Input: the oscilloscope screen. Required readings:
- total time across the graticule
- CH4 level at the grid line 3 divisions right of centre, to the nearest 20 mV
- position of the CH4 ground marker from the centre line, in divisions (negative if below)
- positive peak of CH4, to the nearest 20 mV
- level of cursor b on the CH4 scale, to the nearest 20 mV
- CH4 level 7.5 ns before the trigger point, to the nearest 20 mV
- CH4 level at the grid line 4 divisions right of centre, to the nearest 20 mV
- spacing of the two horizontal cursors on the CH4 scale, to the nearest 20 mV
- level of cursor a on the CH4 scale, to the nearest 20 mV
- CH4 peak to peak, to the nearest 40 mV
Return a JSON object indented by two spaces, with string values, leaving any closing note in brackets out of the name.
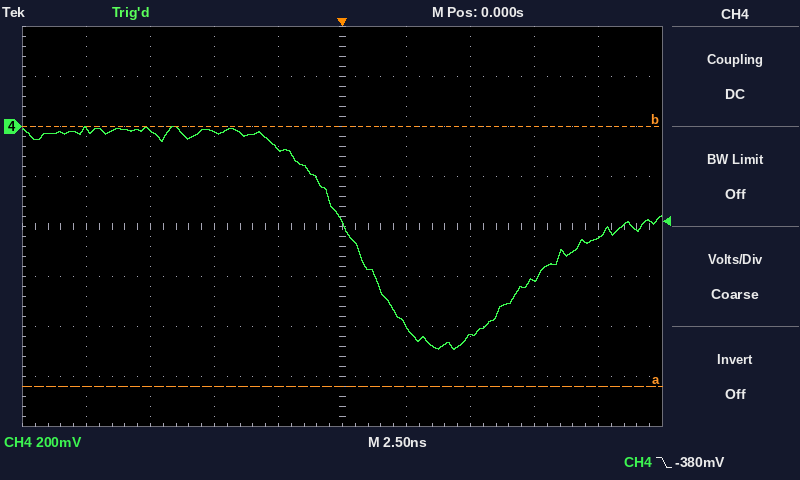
{
  "total time across the graticule": "25 ns",
  "CH4 level at the grid line 3 divisions right of centre, to the nearest 20 mV": "-620 mV",
  "position of the CH4 ground marker from the centre line, in divisions": "+2.0 div",
  "positive peak of CH4, to the nearest 20 mV": "0 mV",
  "level of cursor b on the CH4 scale, to the nearest 20 mV": "0 mV",
  "CH4 level 7.5 ns before the trigger point, to the nearest 20 mV": "-20 mV",
  "CH4 level at the grid line 4 divisions right of centre, to the nearest 20 mV": "-440 mV",
  "spacing of the two horizontal cursors on the CH4 scale, to the nearest 20 mV": "1.04 V",
  "level of cursor a on the CH4 scale, to the nearest 20 mV": "-1.04 V",
  "CH4 peak to peak, to the nearest 40 mV": "880 mV"
}
